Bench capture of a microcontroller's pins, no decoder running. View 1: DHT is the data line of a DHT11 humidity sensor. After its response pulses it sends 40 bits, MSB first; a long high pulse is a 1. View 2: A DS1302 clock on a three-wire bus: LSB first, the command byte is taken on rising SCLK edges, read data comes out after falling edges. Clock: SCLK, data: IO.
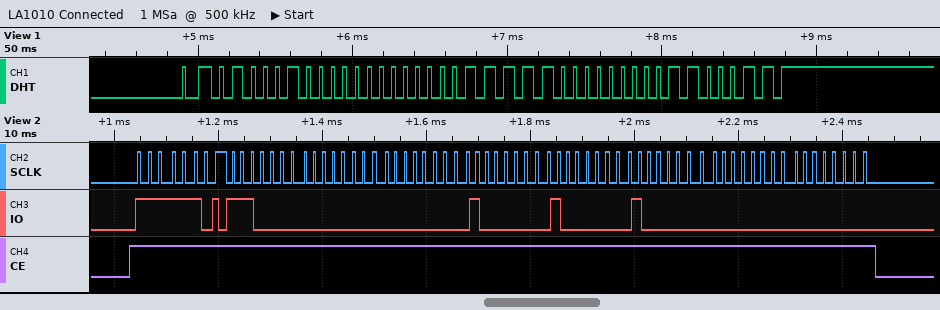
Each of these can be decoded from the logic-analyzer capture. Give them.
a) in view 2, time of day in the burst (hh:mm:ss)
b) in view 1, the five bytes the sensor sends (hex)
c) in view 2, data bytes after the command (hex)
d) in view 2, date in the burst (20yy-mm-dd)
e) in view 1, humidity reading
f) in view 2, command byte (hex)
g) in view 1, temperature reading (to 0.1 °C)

00:00:07
44 00 1F 00 63
07 00 00 01 01 01 00 00
2000-01-01
68 %
0xBF
31.0 °C
